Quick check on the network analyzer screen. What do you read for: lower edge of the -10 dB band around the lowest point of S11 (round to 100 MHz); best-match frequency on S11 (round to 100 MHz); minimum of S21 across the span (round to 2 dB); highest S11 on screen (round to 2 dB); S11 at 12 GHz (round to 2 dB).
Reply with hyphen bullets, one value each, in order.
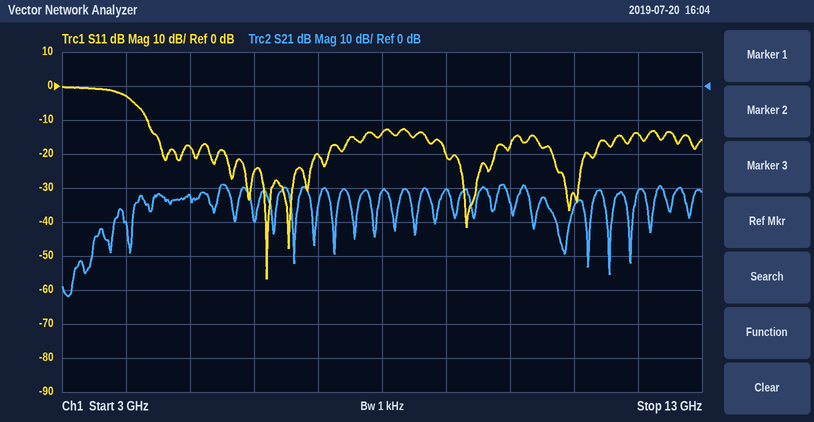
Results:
- 4.3 GHz
- 6.2 GHz
- -62 dB
- 0 dB
- -14 dB
